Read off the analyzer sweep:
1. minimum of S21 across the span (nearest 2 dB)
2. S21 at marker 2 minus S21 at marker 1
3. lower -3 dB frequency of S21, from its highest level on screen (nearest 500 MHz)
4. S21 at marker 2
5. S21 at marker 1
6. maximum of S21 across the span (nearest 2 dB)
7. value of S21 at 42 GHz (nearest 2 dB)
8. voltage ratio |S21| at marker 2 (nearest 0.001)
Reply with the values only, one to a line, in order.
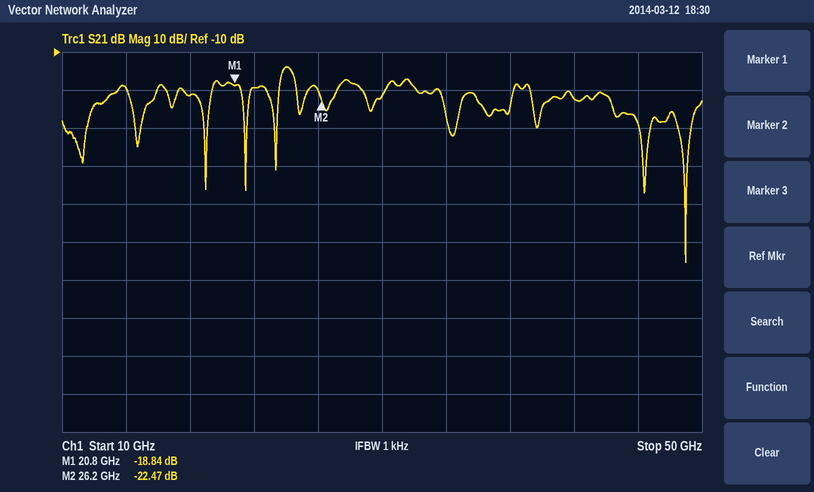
-66 dB
-3.63 dB
23.5 GHz
-22.47 dB
-18.84 dB
-14 dB
-22 dB
0.075
